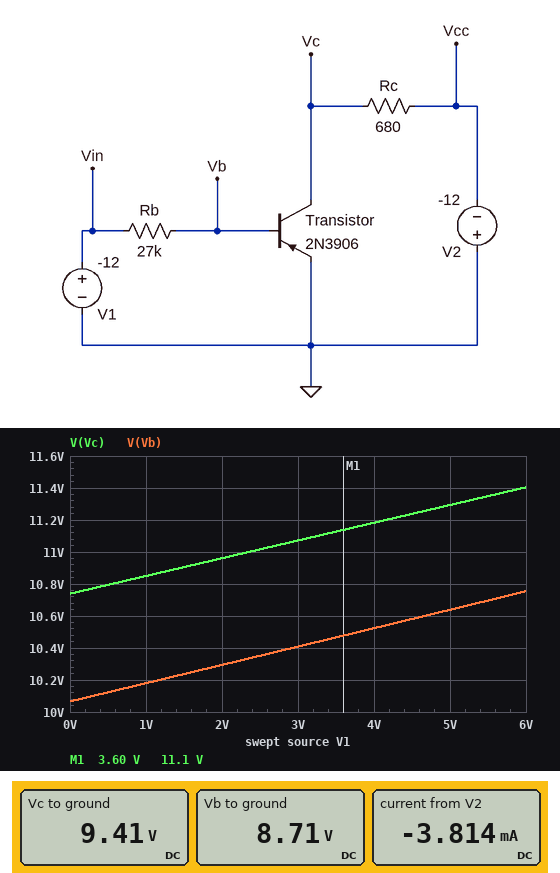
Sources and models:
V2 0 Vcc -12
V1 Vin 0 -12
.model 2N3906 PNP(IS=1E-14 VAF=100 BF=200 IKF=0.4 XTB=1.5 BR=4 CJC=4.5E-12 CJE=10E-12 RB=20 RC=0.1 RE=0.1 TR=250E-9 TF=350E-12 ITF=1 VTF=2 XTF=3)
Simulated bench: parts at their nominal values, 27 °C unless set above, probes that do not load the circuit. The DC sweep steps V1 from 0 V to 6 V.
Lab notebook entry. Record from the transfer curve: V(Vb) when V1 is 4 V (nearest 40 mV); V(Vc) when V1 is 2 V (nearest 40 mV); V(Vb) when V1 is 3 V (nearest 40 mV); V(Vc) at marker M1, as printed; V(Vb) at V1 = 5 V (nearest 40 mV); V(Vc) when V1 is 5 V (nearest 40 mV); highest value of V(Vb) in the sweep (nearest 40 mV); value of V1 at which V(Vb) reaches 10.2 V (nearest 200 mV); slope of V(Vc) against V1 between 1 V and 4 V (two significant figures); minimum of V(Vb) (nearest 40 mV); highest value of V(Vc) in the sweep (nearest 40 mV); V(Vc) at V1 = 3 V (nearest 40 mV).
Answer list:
10.52 V
10.96 V
10.40 V
11.1 V
10.64 V
11.28 V
10.76 V
1.2 V
0.11 V/V
10.08 V
11.40 V
11.08 V
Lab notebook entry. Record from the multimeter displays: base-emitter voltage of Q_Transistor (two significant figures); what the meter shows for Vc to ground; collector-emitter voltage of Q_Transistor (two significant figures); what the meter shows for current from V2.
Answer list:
8.7 V
9.41 V
9.4 V
-3.814 mA
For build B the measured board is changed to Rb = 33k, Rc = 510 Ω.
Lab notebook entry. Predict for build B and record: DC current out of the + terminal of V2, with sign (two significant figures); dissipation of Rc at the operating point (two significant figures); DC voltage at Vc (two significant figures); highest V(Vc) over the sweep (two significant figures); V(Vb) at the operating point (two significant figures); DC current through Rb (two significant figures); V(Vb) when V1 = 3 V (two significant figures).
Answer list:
-3.3 mA
5.4 mW
10 V
12 V
9.6 V
660 µA
11 V
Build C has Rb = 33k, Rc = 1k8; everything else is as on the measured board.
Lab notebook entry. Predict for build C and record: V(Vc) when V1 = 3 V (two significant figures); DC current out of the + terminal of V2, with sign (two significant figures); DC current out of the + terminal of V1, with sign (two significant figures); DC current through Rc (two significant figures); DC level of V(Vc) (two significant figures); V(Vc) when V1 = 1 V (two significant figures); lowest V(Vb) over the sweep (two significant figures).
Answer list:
10 V
-2.8 mA
-560 µA
2.8 mA
7.0 V
9.8 V
8.9 V
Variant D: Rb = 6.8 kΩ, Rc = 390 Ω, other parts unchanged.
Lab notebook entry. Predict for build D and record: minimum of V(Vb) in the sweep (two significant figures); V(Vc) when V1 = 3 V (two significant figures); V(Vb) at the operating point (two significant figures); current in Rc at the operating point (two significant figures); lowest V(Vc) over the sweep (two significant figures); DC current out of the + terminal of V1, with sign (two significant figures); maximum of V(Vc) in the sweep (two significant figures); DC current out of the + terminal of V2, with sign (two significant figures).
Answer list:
8.8 V
10 V
6.1 V
13 mA
9.5 V
-2.7 mA
11 V
-13 mA
